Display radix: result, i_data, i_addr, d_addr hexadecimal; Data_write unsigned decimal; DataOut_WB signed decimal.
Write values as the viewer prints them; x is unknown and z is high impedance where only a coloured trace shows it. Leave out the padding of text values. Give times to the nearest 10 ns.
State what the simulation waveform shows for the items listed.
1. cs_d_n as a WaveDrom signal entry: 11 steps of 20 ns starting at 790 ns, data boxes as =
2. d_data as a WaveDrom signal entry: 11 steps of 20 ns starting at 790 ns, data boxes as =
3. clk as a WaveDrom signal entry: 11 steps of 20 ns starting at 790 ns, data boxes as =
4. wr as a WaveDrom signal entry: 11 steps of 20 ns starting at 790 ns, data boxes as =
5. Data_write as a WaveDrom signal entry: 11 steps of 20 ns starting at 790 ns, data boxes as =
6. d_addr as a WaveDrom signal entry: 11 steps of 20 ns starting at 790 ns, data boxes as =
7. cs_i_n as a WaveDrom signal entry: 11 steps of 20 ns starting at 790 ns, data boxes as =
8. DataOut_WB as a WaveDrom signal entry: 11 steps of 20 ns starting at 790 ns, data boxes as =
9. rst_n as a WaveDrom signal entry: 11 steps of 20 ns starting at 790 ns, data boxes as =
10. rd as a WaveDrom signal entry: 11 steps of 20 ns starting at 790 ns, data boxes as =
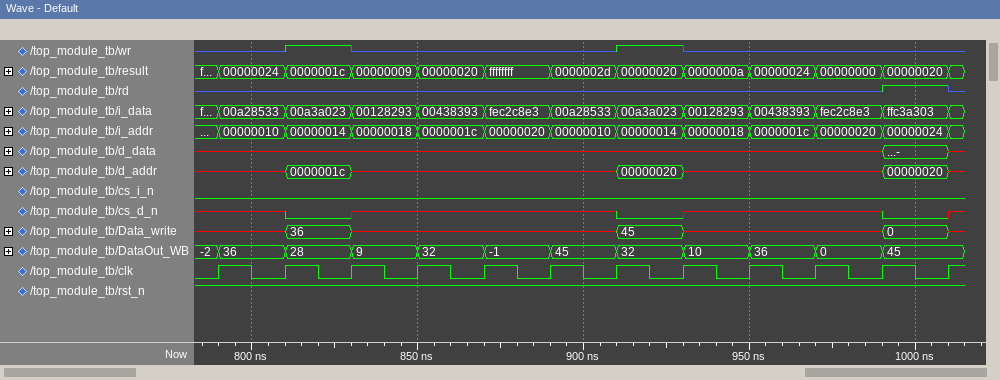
{name: 'cs_d_n', wave: 'x0x...0x..0'}
{name: 'd_data', wave: 'x.........=', data: '-'}
{name: 'clk', wave: 'p..........'}
{name: 'wr', wave: 'z1z...1z...'}
{name: 'Data_write', wave: 'x=x...=x..=', data: '36 45 0'}
{name: 'd_addr', wave: 'x=x...=x..=', data: '0000001c 00000020 00000020'}
{name: 'cs_i_n', wave: '0..........'}
{name: 'DataOut_WB', wave: '===========', data: '36 28 9 32 -1 45 32 10 36 0 45'}
{name: 'rst_n', wave: '1..........'}
{name: 'rd', wave: 'z.........1'}
